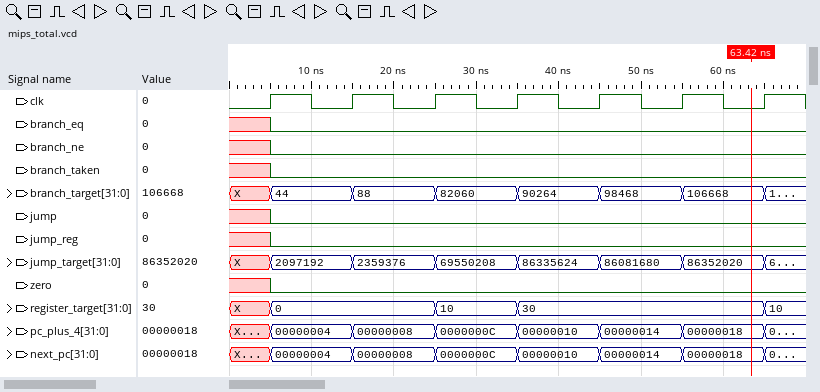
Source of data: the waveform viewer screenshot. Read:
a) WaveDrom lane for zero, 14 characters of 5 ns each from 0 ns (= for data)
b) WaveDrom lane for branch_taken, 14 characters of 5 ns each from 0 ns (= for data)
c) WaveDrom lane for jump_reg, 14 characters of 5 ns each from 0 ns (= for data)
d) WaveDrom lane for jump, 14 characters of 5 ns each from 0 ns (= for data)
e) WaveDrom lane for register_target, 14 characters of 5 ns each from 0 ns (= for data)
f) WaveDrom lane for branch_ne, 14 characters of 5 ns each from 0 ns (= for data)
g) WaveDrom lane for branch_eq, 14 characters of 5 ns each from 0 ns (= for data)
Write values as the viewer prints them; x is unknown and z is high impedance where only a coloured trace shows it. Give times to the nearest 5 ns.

{name: 'zero', wave: 'x0............'}
{name: 'branch_taken', wave: 'x0............'}
{name: 'jump_reg', wave: 'x0............'}
{name: 'jump', wave: 'x0............'}
{name: 'register_target', wave: 'x=...=.=.....=', data: '0 10 30 10'}
{name: 'branch_ne', wave: 'x0............'}
{name: 'branch_eq', wave: 'x0............'}
